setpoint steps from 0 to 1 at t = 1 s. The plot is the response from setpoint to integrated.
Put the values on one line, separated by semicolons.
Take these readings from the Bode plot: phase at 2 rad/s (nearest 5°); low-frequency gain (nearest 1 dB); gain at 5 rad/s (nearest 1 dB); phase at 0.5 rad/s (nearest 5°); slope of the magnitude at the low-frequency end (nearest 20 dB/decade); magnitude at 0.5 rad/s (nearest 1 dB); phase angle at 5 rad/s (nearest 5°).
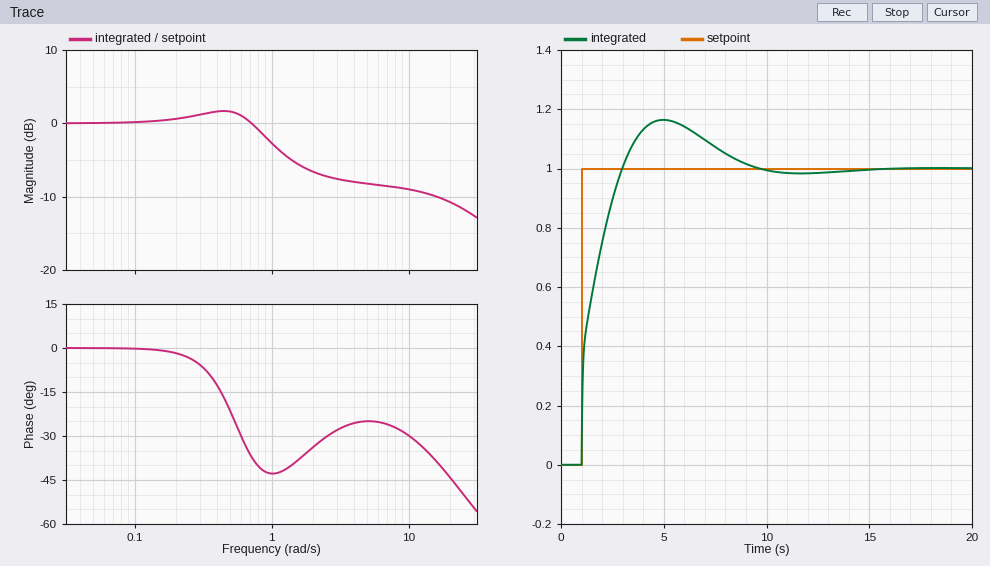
-35°; 0 dB; -8 dB; -20°; 0 dB/decade; 2 dB; -25°
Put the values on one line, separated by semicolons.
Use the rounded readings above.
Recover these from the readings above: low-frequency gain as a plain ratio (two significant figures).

1.0
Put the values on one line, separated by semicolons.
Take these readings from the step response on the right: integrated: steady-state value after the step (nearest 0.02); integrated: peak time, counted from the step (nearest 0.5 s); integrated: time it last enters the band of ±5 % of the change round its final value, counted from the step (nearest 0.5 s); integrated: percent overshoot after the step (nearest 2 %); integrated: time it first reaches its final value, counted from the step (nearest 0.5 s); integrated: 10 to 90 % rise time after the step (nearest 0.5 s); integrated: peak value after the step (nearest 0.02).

1.00; 4.0 s; 7.0 s; 16 %; 2.0 s; 1.5 s; 1.16
